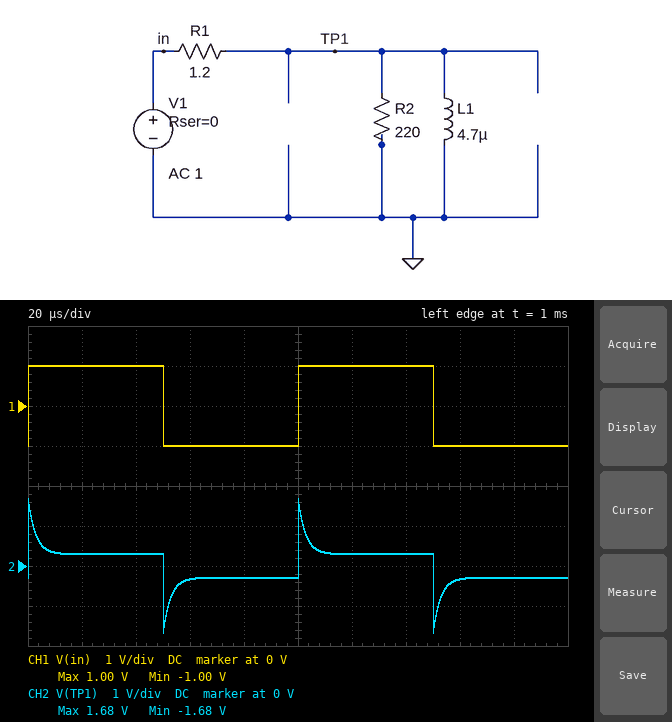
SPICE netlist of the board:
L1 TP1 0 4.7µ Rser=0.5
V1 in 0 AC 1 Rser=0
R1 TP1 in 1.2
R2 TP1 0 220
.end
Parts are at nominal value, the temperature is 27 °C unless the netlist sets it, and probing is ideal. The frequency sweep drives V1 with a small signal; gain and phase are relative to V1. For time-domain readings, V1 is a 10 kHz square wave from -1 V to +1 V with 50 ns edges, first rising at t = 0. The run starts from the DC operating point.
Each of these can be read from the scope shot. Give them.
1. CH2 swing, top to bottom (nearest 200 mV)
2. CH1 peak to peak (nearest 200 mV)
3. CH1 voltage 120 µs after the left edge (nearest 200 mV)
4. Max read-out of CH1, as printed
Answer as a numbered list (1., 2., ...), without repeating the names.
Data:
1. 3.4 V
2. 2.0 V
3. 1.0 V
4. 1.00 V
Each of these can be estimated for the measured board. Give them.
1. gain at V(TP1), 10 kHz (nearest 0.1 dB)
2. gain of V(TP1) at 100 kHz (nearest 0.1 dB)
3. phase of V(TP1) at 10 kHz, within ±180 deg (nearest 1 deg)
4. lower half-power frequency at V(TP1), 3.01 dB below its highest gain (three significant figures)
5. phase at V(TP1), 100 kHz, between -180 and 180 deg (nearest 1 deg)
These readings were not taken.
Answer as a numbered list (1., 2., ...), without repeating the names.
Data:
1. -9.5 dB
2. -1.2 dB
3. 21 deg
4. 52.1 kHz
5. 20 deg
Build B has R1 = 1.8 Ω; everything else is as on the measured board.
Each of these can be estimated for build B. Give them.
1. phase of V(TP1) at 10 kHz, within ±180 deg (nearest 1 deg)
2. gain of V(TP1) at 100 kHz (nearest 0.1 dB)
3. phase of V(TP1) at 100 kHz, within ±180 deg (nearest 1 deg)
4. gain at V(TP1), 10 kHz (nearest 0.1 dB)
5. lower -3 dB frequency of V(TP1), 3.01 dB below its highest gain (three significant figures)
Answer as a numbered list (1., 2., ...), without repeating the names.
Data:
1. 23 deg
2. -2.0 dB
3. 28 deg
4. -12.0 dB
5. 73.6 kHz
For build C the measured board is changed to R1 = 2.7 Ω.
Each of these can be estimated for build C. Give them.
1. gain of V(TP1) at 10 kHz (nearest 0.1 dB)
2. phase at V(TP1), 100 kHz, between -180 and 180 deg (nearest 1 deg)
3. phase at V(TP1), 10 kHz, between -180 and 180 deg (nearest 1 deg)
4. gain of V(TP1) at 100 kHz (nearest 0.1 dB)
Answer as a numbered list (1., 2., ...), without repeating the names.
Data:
1. -14.9 dB
2. 37 deg
3. 25 deg
4. -3.3 dB
